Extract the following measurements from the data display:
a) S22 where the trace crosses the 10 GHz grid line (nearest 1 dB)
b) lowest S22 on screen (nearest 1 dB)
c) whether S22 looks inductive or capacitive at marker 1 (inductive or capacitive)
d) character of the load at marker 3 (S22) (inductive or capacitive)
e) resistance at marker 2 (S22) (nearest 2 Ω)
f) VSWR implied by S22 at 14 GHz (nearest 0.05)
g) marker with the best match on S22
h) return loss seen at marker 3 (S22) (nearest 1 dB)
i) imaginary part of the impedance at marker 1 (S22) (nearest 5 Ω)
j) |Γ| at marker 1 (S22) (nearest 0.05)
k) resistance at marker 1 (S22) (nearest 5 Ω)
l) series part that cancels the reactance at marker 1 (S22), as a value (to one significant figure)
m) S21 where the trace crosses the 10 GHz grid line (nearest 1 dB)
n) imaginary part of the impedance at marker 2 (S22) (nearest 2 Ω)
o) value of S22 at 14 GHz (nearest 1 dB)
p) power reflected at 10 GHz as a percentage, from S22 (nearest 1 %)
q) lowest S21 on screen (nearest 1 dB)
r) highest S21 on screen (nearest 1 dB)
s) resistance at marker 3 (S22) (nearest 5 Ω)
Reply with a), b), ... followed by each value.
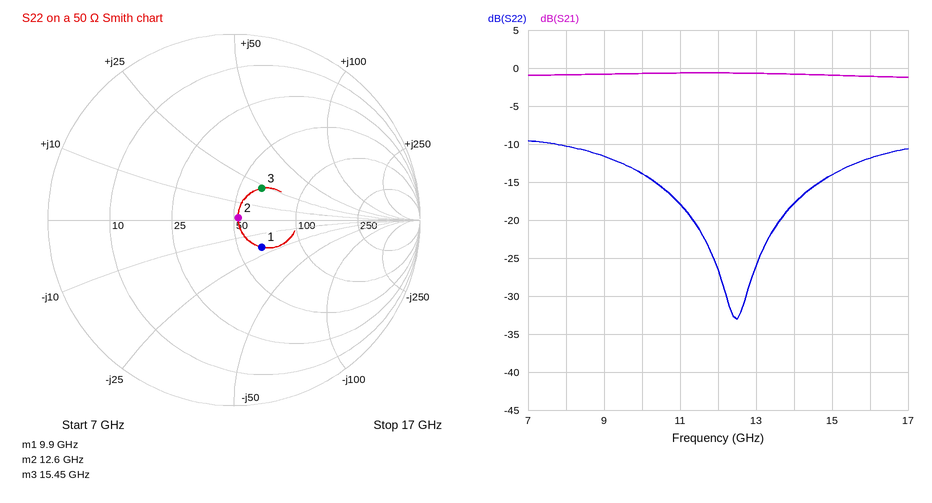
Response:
a) -14 dB
b) -33 dB
c) capacitive
d) inductive
e) 52 Ω
f) 1.30
g) marker 2
h) 13 dB
i) -20 Ω
j) 0.20
k) 65 Ω
l) 300 pH
m) -1 dB
n) +2 Ω
o) -18 dB
p) 4 %
q) -1 dB
r) -1 dB
s) 65 Ω
